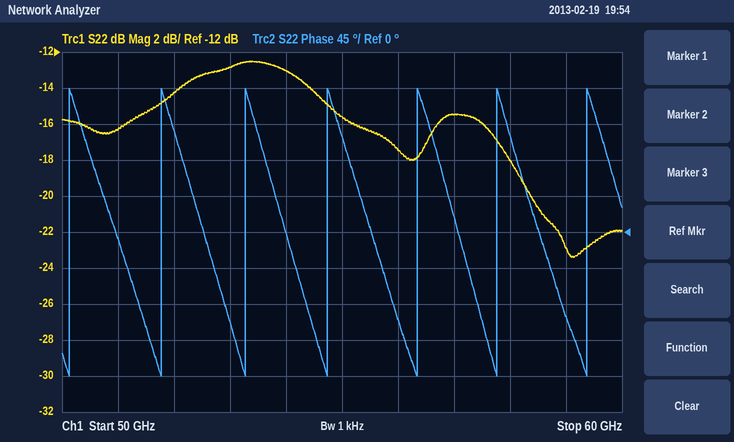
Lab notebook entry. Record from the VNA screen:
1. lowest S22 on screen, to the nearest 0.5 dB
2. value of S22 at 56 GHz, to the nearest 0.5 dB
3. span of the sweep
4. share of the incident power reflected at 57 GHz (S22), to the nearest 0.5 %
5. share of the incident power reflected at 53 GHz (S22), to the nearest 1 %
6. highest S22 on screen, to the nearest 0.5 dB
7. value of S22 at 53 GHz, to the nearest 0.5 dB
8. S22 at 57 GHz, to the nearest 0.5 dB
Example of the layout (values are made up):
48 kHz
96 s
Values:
-23.5 dB
-17.5 dB
10 GHz
3.0 %
5 %
-12.5 dB
-13.0 dB
-15.5 dB
